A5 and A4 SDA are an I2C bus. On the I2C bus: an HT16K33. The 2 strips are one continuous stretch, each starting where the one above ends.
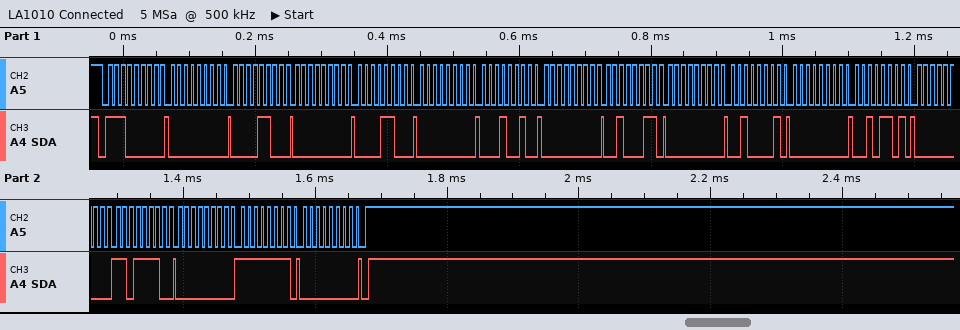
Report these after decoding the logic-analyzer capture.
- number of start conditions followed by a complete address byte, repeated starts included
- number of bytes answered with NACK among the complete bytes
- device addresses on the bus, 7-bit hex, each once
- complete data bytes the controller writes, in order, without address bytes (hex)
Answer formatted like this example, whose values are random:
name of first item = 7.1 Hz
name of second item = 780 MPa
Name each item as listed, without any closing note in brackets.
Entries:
number of start conditions followed by a complete address byte, repeated starts included = 1
number of bytes answered with NACK among the complete bytes = 0
device addresses on the bus, 7-bit hex, each once = 0x70
complete data bytes the controller writes, in order, without address bytes = 00 0C 00 0C 00 12 00 23 00 21 00 2D 00 DE 00 FF 00
